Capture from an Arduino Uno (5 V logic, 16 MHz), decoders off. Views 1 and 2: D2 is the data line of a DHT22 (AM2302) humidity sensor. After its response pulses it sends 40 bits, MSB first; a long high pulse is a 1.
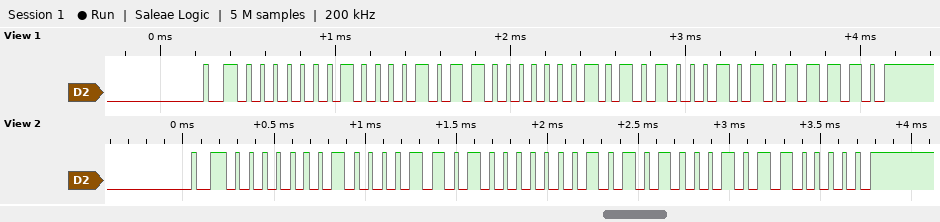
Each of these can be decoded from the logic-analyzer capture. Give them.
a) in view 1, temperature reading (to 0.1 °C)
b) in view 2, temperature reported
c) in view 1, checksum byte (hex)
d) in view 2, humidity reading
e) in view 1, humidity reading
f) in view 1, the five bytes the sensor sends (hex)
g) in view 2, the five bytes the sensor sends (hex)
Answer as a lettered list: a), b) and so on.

a) 33.7 °C
b) 33.7 °C
c) 0x5E
d) 26.9 %
e) 26.7 %
f) 01 0B 01 51 5E
g) 01 0D 01 51 60
